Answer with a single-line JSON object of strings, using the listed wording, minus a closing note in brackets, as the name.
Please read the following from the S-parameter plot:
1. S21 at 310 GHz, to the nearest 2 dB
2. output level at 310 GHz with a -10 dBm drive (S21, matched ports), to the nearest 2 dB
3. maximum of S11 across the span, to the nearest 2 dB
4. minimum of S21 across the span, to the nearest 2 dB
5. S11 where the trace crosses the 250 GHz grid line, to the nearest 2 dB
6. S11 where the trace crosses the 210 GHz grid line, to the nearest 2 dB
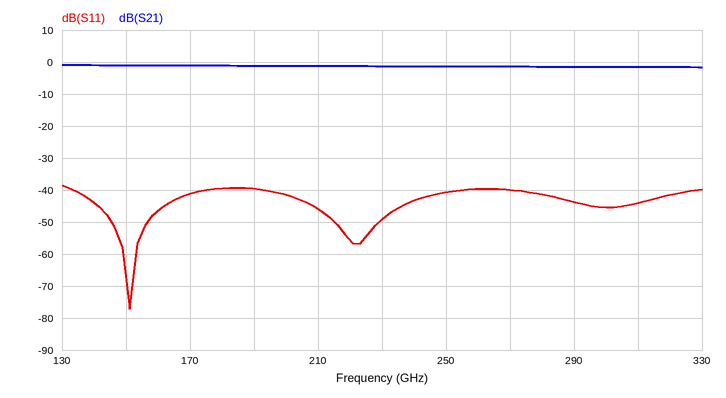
{"S21 at 310 GHz, to the nearest 2 dB": "-2 dB", "output level at 310 GHz with a -10 dBm drive (S21, matched ports), to the nearest 2 dB": "-12 dBm", "maximum of S11 across the span, to the nearest 2 dB": "-38 dB", "minimum of S21 across the span, to the nearest 2 dB": "-2 dB", "S11 where the trace crosses the 250 GHz grid line, to the nearest 2 dB": "-40 dB", "S11 where the trace crosses the 210 GHz grid line, to the nearest 2 dB": "-46 dB"}
